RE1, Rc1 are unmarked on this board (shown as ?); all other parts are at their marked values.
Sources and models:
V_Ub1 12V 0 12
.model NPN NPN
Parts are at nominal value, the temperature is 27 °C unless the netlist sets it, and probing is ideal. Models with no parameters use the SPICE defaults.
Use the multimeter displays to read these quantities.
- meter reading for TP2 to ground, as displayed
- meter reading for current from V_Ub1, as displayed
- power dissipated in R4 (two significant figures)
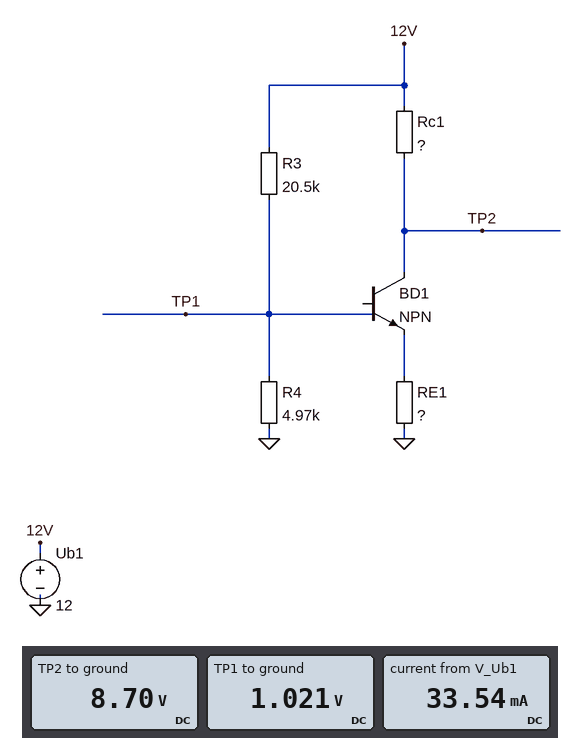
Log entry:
8.70 V
33.54 mA
210 µW
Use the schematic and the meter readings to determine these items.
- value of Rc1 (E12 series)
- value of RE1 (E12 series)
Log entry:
100 Ω
4.7 Ω
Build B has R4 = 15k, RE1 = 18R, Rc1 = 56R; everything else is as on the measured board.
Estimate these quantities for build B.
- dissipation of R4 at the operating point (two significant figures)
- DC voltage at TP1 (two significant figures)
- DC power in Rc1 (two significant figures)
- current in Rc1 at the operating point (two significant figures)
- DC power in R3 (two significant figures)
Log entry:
170 µW
1.6 V
90 mW
40 mA
5.3 mW
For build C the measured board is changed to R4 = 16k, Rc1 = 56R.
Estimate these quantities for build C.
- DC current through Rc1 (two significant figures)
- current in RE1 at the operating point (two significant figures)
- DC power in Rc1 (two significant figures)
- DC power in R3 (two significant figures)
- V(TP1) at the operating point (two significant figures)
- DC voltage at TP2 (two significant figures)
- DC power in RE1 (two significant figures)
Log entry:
46 mA
47 mA
120 mW
5.8 mW
1.1 V
9.4 V
10 mW
